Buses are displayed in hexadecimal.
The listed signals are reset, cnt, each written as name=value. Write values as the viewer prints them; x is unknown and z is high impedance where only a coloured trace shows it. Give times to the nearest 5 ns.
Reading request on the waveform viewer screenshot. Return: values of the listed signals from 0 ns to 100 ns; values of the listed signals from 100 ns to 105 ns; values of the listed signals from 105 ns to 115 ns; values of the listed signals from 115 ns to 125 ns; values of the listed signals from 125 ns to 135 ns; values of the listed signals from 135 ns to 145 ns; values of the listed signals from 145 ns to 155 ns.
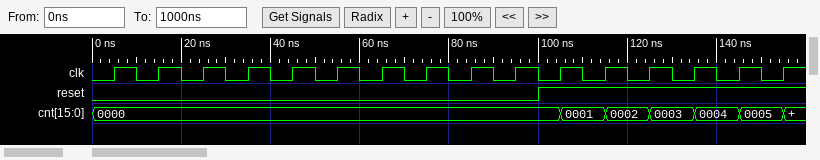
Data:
reset=0, cnt=0000
reset=1, cnt=0000
reset=1, cnt=0001
reset=1, cnt=0002
reset=1, cnt=0003
reset=1, cnt=0004
reset=1, cnt=0005
